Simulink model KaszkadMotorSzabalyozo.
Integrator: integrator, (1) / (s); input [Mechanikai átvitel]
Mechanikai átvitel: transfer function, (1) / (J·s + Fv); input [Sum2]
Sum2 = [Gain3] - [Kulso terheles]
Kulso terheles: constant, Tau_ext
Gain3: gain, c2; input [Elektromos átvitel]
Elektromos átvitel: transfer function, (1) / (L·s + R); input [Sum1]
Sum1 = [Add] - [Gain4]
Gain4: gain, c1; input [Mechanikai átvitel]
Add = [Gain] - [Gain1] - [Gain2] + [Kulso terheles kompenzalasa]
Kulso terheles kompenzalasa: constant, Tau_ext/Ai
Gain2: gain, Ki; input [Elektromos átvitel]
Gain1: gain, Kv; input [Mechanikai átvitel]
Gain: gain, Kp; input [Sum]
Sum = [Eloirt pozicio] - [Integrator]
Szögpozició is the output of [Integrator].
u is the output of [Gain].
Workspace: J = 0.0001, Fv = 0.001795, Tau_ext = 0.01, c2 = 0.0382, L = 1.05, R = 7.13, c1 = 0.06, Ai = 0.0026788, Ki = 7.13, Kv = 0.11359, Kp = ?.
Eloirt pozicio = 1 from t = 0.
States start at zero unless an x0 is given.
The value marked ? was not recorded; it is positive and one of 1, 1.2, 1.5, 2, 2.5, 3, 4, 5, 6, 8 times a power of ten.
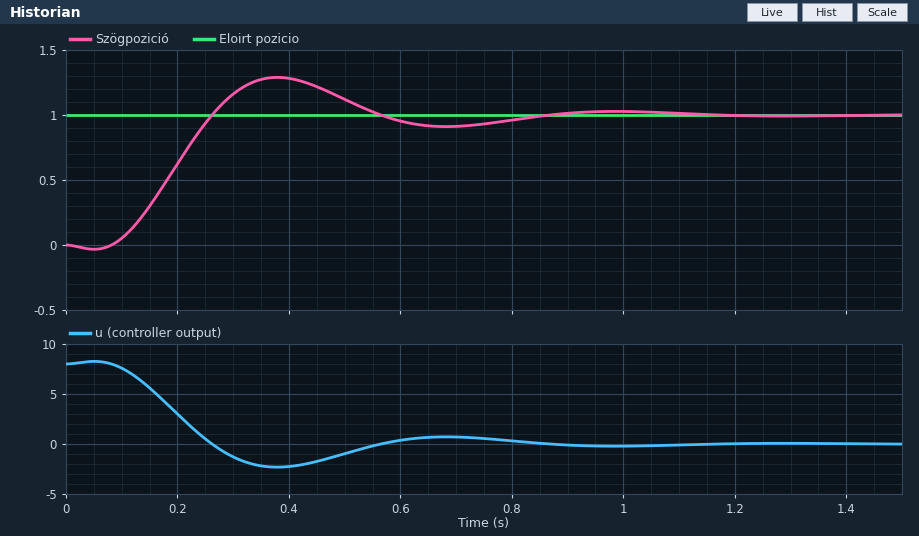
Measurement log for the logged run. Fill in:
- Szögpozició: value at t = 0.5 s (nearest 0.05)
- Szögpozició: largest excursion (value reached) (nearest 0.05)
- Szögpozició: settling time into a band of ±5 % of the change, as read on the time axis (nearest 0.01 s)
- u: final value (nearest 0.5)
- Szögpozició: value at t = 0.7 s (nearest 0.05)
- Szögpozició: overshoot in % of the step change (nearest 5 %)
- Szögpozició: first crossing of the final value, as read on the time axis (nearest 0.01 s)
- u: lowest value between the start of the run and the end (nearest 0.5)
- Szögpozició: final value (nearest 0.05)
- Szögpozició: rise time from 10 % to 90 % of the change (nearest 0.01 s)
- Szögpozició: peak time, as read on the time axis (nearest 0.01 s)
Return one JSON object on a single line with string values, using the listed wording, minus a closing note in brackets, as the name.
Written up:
{"Szögpozició: value at t = 0.5 s": "1.10", "Szögpozició: largest excursion (value reached)": "1.30", "Szögpozició: settling time into a band of ±5 % of the change, as read on the time axis": "0.78 s", "u: final value": "0.0", "Szögpozició: value at t = 0.7 s": "0.90", "Szögpozició: overshoot in % of the step change": "30 %", "Szögpozició: first crossing of the final value, as read on the time axis": "0.26 s", "u: lowest value between the start of the run and the end": "-2.5", "Szögpozició: final value": "1.00", "Szögpozició: rise time from 10 % to 90 % of the change": "0.13 s", "Szögpozició: peak time, as read on the time axis": "0.38 s"}
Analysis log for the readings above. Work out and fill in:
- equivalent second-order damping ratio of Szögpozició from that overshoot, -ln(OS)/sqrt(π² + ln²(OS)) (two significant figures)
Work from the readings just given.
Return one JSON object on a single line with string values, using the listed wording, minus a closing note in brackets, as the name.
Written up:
{"equivalent second-order damping ratio of Szögpozició from that overshoot, -ln(OS)/sqrt(π² + ln²(OS))": "0.36"}
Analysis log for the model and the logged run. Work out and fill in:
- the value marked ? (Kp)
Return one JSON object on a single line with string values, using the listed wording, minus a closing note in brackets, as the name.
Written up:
{"the value marked ?": "8"}
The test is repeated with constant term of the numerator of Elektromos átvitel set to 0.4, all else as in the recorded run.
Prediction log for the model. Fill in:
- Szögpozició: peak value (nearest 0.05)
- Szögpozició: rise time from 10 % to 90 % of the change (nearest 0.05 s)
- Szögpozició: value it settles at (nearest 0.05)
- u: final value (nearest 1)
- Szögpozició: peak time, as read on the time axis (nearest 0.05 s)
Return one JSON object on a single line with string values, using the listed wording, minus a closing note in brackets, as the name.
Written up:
{"Szögpozició: peak value": "0.80", "Szögpozició: rise time from 10 % to 90 % of the change": "0.15 s", "Szögpozició: value it settles at": "0.65", "u: final value": "3", "Szögpozició: peak time, as read on the time axis": "0.60 s"}
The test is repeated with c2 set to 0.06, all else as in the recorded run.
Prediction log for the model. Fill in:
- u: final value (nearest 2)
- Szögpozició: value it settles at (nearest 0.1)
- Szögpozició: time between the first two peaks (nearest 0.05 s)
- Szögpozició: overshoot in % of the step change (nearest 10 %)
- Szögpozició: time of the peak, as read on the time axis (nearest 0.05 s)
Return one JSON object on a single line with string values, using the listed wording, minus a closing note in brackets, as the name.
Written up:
{"u: final value": "-2", "Szögpozició: value it settles at": "1.2", "Szögpozició: time between the first two peaks": "0.50 s", "Szögpozició: overshoot in % of the step change": "40 %", "Szögpozició: time of the peak, as read on the time axis": "0.30 s"}
